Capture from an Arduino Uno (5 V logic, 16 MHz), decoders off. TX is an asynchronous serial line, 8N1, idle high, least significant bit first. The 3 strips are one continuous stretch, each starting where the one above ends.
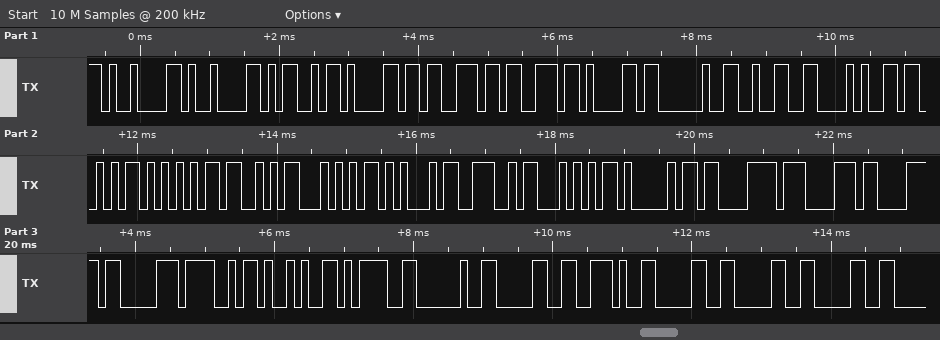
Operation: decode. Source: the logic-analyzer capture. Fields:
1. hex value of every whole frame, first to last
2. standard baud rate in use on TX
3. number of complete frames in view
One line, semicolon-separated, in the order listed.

09 09 4D 61 73 73 61 20 32 28 53 55 53 54 45 4E 54 41 C3 87 C3 83 4F 29 3D 20 30 2E 30 30 30; 9600 baud; 31
